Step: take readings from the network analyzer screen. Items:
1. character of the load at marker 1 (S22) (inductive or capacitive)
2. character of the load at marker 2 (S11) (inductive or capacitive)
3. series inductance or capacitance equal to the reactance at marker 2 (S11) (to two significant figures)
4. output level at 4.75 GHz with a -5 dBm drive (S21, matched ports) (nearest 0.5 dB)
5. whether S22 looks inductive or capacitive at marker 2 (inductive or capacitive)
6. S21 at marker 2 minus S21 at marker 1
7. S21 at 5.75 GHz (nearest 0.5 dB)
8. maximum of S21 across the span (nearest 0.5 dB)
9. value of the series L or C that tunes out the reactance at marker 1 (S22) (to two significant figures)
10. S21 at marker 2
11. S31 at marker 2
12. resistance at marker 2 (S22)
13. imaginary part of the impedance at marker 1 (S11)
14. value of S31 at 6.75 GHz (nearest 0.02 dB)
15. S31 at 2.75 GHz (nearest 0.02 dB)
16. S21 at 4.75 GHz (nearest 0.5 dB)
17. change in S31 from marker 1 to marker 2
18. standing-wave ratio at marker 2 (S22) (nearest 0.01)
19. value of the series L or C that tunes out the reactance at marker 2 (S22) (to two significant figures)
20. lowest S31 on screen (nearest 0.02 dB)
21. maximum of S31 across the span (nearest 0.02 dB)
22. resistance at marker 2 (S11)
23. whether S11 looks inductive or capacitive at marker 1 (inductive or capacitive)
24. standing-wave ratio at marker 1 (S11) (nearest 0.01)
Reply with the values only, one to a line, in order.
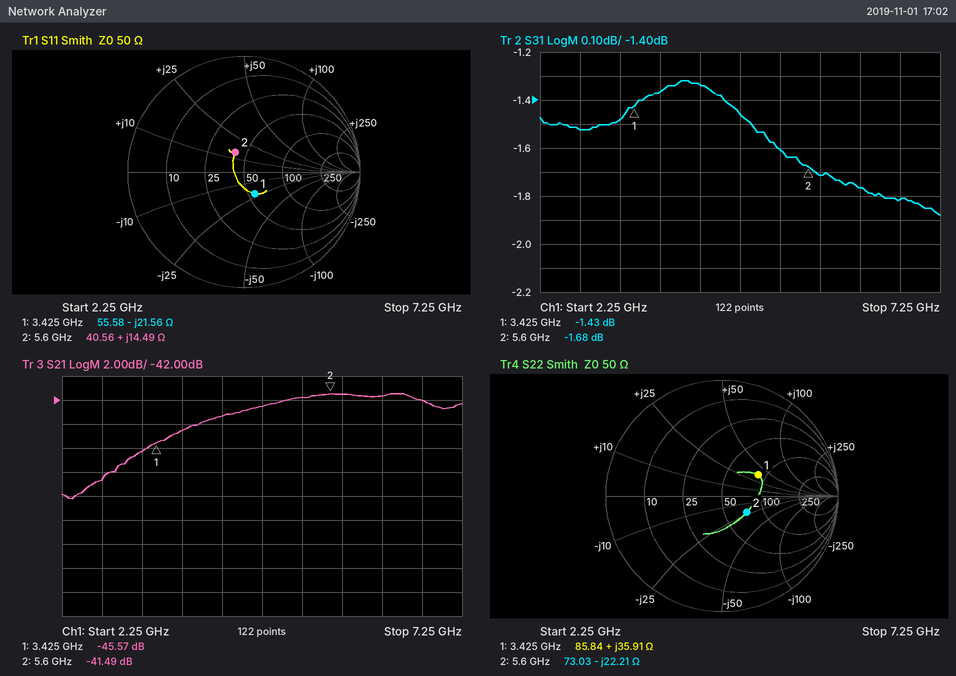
inductive
inductive
410 pH
-47.5 dBm
capacitive
4.08 dB
-41.5 dB
-41.5 dB
1.3 pF
-41.49 dB
-1.68 dB
73.03 Ω
-21.56 Ω
-1.82 dB
-1.52 dB
-42.5 dB
-0.25 dB
1.69
630 pH
-1.88 dB
-1.32 dB
40.56 Ω
capacitive
1.52
